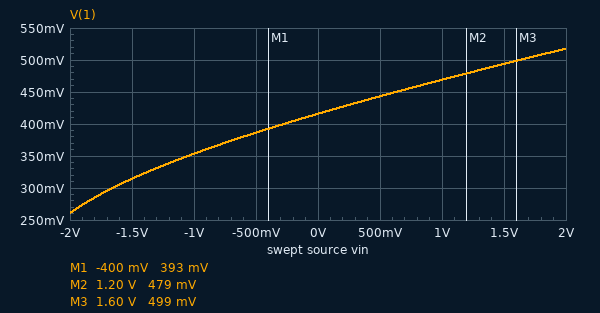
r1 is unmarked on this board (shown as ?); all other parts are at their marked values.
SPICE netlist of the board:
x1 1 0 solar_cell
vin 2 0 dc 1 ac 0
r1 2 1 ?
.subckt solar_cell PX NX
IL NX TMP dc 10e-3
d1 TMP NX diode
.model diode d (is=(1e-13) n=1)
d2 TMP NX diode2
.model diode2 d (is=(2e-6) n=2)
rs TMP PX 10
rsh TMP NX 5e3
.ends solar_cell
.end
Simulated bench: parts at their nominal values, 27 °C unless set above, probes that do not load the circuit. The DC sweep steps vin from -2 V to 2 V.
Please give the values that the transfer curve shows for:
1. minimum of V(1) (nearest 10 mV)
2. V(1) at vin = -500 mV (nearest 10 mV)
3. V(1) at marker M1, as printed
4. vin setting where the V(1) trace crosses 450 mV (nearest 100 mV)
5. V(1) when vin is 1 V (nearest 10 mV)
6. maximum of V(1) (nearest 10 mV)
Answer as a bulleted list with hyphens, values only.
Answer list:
- 260 mV
- 390 mV
- 393 mV
- 600 mV
- 470 mV
- 520 mV
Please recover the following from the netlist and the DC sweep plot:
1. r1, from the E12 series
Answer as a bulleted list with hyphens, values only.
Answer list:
- 270 Ω
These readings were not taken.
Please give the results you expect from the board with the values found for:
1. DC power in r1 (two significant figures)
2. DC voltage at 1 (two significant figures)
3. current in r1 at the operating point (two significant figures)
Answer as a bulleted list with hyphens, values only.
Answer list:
- 1.0 mW
- 470 mV
- 2.0 mA
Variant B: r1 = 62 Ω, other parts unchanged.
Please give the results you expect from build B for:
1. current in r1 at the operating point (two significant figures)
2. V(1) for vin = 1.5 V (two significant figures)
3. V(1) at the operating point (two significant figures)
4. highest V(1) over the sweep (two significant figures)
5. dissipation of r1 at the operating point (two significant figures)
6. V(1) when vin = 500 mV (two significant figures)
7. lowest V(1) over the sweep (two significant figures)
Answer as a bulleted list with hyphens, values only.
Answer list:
- 7.4 mA
- 630 mV
- 540 mV
- 710 mV
- 3.4 mW
- 450 mV
- -1.4 V
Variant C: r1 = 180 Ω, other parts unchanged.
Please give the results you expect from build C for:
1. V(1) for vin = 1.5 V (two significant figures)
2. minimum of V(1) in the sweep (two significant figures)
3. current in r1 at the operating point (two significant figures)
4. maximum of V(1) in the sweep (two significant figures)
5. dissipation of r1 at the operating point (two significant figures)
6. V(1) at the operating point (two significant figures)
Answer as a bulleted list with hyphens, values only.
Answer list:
- 520 mV
- -200 mV
- 2.9 mA
- 550 mV
- 1.5 mW
- 480 mV
